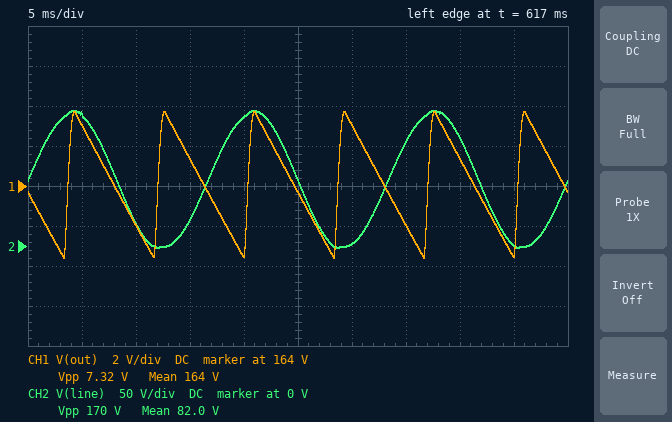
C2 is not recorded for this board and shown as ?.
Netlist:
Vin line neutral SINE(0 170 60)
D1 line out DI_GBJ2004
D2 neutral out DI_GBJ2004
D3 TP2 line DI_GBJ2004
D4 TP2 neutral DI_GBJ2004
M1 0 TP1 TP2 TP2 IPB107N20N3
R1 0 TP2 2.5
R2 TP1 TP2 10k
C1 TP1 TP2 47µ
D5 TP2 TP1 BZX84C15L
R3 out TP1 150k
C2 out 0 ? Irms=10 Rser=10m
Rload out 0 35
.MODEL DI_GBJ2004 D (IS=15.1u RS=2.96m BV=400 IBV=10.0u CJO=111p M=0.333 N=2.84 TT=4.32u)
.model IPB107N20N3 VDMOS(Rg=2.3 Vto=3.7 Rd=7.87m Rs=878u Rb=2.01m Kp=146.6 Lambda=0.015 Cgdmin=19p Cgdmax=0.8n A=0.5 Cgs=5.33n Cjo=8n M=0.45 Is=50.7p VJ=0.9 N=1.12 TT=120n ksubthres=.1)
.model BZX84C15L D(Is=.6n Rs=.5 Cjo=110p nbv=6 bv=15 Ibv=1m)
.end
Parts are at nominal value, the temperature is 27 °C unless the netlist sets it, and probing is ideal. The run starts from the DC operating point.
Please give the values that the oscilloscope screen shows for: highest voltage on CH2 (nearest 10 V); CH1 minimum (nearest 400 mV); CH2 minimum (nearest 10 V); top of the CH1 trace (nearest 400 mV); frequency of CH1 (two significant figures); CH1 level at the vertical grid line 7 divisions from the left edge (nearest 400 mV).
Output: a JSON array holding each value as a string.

["170 V", "160.4 V", "0 V", "167.6 V", "120 Hz", "162.0 V"]
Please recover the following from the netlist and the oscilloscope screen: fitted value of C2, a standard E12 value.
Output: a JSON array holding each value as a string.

["4.7 mF"]
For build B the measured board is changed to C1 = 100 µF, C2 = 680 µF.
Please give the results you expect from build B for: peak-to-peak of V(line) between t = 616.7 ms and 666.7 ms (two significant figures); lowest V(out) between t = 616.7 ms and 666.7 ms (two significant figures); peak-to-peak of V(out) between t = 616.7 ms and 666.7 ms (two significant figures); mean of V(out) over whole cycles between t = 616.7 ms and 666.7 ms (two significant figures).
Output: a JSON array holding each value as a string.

["170 V", "130 V", "39 V", "150 V"]
